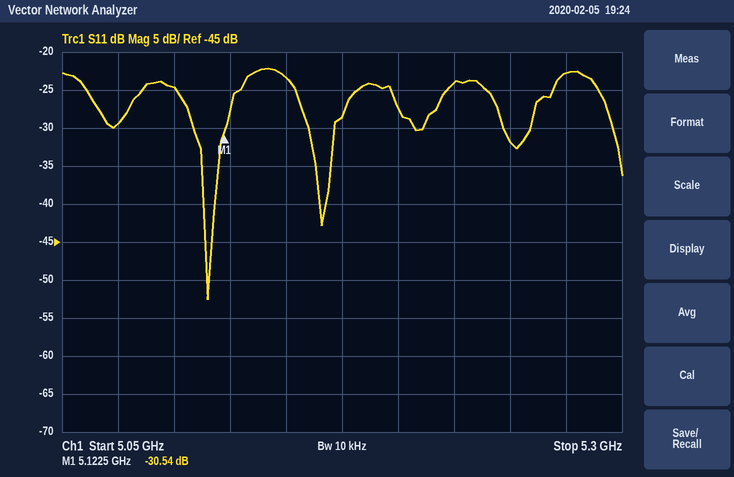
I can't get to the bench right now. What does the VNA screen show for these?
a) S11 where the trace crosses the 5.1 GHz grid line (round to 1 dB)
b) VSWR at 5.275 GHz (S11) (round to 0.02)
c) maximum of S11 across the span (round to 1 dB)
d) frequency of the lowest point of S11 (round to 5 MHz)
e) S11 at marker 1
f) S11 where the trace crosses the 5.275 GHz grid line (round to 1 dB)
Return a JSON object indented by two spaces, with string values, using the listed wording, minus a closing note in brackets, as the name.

{
  "S11 where the trace crosses the 5.1 GHz grid line": "-25 dB",
  "VSWR at 5.275 GHz (S11)": "1.16",
  "maximum of S11 across the span": "-22 dB",
  "frequency of the lowest point of S11": "5.115 GHz",
  "S11 at marker 1": "-30.54 dB",
  "S11 where the trace crosses the 5.275 GHz grid line": "-23 dB"
}
